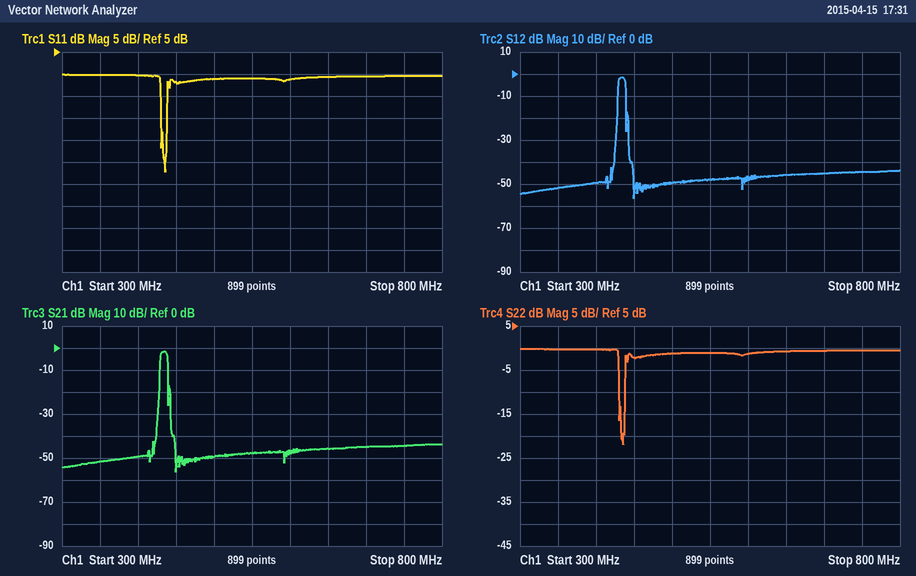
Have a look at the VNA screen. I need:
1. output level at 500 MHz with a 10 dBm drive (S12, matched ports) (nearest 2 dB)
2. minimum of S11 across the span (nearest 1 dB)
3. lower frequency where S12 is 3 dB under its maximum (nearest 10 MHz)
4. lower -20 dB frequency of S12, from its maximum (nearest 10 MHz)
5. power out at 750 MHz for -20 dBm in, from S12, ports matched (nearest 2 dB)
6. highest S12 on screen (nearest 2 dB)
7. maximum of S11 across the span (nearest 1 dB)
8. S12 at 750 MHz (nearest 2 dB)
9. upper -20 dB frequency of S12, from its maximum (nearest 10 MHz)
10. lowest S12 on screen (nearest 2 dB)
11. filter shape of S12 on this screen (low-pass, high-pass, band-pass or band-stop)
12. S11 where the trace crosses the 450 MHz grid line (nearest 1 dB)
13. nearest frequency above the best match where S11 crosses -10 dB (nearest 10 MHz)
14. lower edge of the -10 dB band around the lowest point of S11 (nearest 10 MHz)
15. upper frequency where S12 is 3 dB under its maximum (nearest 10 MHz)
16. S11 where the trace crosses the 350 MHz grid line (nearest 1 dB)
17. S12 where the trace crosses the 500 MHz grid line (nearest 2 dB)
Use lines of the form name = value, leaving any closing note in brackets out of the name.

output level at 500 MHz with a 10 dBm drive (S12, matched ports) = -40 dBm
minimum of S11 across the span = -22 dB
lower frequency where S12 is 3 dB under its maximum = 430 MHz
lower -20 dB frequency of S12, from its maximum = 430 MHz
power out at 750 MHz for -20 dBm in, from S12, ports matched = -64 dBm
highest S12 on screen = -2 dB
maximum of S11 across the span = 0 dB
S12 at 750 MHz = -44 dB
upper -20 dB frequency of S12, from its maximum = 440 MHz
lowest S12 on screen = -56 dB
filter shape of S12 on this screen = band-pass
S11 where the trace crosses the 450 MHz grid line = -2 dB
nearest frequency above the best match where S11 crosses -10 dB = 440 MHz
lower edge of the -10 dB band around the lowest point of S11 = 430 MHz
upper frequency where S12 is 3 dB under its maximum = 440 MHz
S11 where the trace crosses the 350 MHz grid line = 0 dB
S12 where the trace crosses the 500 MHz grid line = -50 dB
